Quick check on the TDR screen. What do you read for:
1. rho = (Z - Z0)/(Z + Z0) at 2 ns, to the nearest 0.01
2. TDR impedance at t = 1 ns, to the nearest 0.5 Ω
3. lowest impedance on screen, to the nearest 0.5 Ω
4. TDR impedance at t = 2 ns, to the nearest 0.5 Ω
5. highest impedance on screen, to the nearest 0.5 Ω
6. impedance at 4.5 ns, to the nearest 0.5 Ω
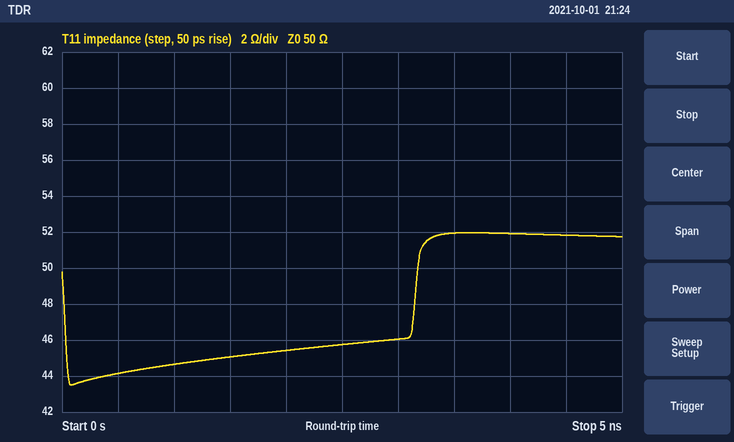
-0.05
44.5 Ω
43.5 Ω
45.5 Ω
52.0 Ω
52.0 Ω
